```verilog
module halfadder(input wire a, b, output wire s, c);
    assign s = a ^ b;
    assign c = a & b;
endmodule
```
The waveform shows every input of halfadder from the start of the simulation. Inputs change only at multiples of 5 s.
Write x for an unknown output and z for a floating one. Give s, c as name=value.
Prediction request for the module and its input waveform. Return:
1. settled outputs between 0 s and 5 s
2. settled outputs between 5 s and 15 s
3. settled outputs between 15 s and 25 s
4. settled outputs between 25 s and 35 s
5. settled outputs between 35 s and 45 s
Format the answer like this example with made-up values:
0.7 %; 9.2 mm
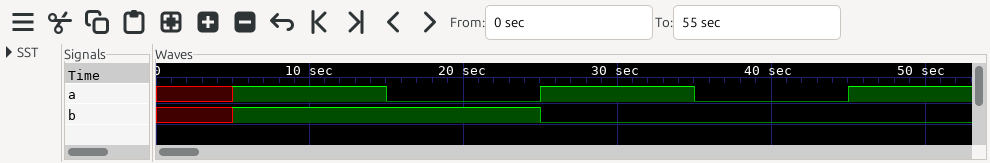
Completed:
s=x, c=x; s=0, c=1; s=1, c=0; s=1, c=0; s=0, c=0
